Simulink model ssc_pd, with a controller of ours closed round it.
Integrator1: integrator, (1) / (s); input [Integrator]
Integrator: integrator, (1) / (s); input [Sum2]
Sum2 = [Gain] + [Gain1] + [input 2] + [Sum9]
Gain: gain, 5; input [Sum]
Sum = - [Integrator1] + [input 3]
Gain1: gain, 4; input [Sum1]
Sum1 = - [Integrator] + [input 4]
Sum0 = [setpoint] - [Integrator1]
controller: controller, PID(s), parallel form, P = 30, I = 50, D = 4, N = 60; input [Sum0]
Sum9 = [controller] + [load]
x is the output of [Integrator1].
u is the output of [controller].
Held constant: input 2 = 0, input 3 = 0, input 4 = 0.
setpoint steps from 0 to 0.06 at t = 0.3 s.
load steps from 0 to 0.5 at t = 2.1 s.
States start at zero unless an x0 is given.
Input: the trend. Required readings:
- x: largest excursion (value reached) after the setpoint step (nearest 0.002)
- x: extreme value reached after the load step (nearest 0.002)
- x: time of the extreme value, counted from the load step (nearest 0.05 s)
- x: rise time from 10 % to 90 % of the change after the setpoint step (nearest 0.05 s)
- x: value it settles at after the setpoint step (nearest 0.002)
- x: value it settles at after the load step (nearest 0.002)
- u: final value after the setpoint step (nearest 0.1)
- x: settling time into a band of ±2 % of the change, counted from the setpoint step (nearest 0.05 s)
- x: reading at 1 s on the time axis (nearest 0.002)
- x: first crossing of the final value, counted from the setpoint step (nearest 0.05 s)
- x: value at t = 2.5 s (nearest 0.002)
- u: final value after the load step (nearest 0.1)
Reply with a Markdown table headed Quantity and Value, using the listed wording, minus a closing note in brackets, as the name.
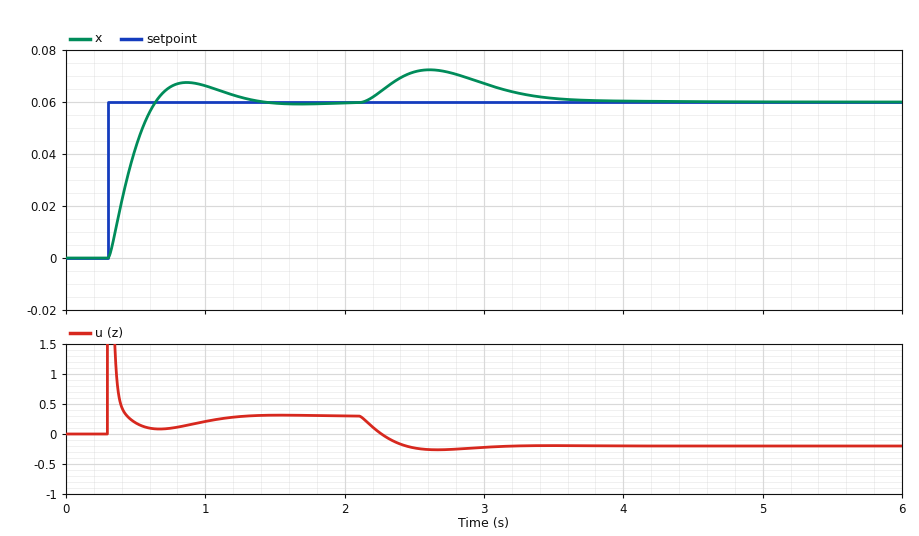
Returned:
| Quantity | Value |
|---|---|
| x: largest excursion (value reached) after the setpoint step | 0.068 |
| x: extreme value reached after the load step | 0.072 |
| x: time of the extreme value, counted from the load step | 0.50 s |
| x: rise time from 10 % to 90 % of the change after the setpoint step | 0.25 s |
| x: value it settles at after the setpoint step | 0.060 |
| x: value it settles at after the load step | 0.060 |
| u: final value after the setpoint step | 0.3 |
| x: settling time into a band of ±2 % of the change, counted from the setpoint step | 1.00 s |
| x: reading at 1 s on the time axis | 0.066 |
| x: first crossing of the final value, counted from the setpoint step | 0.35 s |
| x: value at t = 2.5 s | 0.072 |
| u: final value after the load step | -0.2 |
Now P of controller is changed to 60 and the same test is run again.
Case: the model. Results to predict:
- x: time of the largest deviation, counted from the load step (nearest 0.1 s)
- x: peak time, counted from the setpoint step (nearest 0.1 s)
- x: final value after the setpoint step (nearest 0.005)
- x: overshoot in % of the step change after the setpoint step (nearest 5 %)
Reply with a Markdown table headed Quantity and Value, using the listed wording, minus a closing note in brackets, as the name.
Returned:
| Quantity | Value |
|---|---|
| x: time of the largest deviation, counted from the load step | 0.4 s |
| x: peak time, counted from the setpoint step | 0.4 s |
| x: final value after the setpoint step | 0.060 |
| x: overshoot in % of the step change after the setpoint step | 20 % |
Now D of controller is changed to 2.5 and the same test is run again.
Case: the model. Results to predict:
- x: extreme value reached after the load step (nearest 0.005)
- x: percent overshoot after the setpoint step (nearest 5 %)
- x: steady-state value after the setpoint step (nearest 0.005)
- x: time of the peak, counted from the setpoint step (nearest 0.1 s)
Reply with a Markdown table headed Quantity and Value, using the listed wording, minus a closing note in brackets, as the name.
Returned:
| Quantity | Value |
|---|---|
| x: extreme value reached after the load step | 0.075 |
| x: percent overshoot after the setpoint step | 20 % |
| x: steady-state value after the setpoint step | 0.060 |
| x: time of the peak, counted from the setpoint step | 0.6 s |
